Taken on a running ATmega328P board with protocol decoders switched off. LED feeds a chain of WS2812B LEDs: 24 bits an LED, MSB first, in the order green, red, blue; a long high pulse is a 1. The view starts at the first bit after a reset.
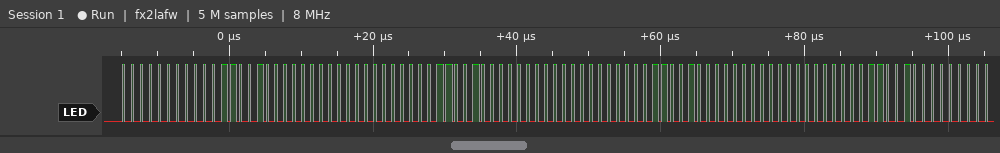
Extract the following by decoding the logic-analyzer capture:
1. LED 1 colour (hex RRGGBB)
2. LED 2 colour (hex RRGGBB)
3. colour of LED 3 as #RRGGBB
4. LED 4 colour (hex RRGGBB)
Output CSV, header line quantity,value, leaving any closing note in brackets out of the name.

quantity,value
LED 1 colour,#190000
LED 2 colour,#190000
colour of LED 3 as #RRGGBB,#190000
LED 4 colour,#190000
